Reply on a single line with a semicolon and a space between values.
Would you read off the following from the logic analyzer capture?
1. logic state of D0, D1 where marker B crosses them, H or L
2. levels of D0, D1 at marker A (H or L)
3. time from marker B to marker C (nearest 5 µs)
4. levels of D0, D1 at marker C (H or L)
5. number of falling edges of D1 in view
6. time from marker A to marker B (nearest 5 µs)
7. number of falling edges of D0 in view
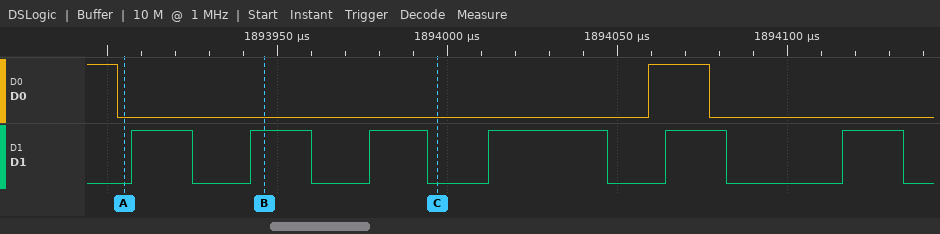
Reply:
D0=L, D1=H; D0=L, D1=L; 50 µs; D0=L, D1=L; 6; 40 µs; 2
